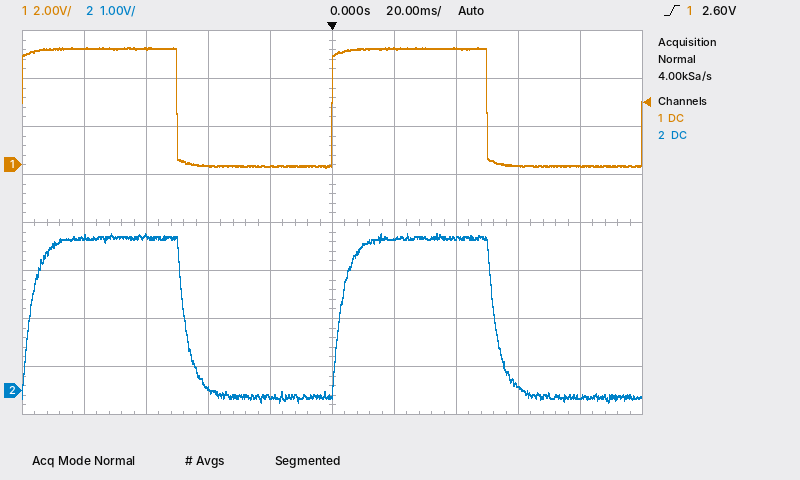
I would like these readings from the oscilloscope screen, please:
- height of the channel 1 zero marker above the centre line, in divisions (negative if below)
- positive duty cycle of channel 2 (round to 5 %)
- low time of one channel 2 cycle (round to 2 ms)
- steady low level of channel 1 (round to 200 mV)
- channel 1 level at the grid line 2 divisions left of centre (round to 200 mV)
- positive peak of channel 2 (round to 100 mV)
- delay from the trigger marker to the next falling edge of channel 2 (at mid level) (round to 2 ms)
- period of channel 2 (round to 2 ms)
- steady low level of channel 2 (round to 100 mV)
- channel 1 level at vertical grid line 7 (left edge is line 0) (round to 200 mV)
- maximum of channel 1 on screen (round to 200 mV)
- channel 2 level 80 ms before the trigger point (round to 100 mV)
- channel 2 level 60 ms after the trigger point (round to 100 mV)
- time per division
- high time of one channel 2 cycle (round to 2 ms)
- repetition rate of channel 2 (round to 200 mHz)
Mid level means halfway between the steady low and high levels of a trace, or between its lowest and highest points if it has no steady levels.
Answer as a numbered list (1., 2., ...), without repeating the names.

1. +1.2 div
2. 50 %
3. 50 ms
4. 0.0 V
5. 0.0 V
6. 3.3 V
7. 52 ms
8. 100 ms
9. -100 mV
10. 4.8 V
11. 4.8 V
12. 3.2 V
13. 100 mV
14. 20 ms
15. 50 ms
16. 10.0 Hz
